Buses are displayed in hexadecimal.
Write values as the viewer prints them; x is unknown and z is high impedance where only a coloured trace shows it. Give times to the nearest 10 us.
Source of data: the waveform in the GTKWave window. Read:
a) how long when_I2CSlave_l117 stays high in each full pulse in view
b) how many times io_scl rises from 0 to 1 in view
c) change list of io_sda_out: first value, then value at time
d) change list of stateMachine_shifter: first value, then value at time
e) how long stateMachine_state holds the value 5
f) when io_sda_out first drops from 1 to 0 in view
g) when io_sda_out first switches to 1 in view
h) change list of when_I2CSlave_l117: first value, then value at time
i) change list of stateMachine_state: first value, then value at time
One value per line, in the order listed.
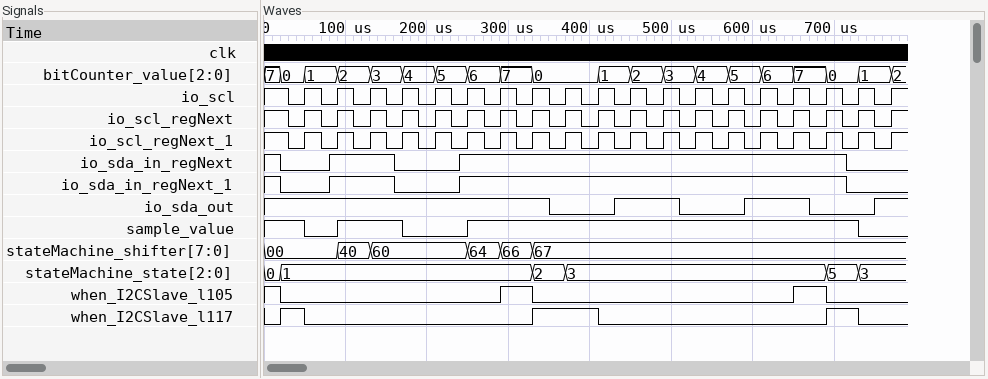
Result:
30 us, 80 us, 40 us
19
1, 0 at 350 us, 1 at 430 us, 0 at 510 us, 1 at 590 us, 0 at 670 us, 1 at 750 us
00, 40 at 90 us, 60 at 130 us, 64 at 250 us, 66 at 290 us, 67 at 330 us
40 us
350 us
430 us
0, 1 at 20 us, 0 at 50 us, 1 at 330 us, 0 at 410 us, 1 at 690 us, 0 at 730 us
0, 1 at 20 us, 2 at 330 us, 3 at 370 us, 5 at 690 us, 3 at 730 us
